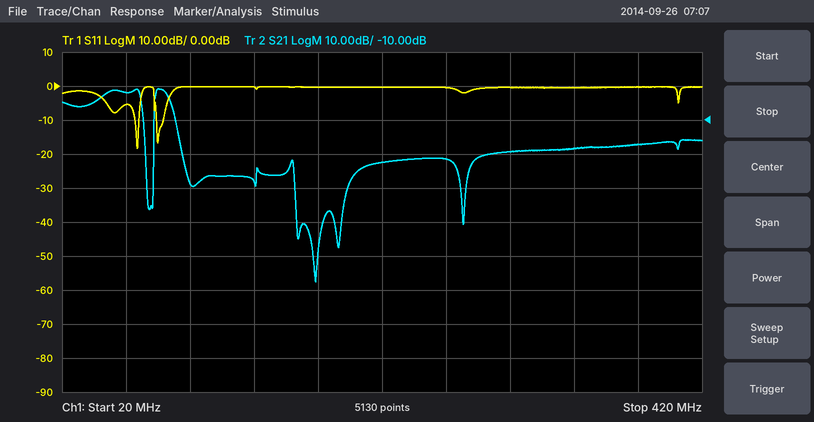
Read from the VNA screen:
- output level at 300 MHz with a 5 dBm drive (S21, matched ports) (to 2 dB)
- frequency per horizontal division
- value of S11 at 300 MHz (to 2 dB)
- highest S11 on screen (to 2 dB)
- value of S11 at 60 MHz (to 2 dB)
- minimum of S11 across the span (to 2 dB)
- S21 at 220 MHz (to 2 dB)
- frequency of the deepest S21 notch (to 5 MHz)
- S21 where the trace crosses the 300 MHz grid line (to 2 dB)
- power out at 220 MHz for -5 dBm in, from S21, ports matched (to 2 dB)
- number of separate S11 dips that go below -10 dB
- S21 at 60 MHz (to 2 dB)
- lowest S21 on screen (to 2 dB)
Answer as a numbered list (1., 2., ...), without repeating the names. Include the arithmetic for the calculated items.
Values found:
1. 5 dBm + (-20 dB) = -14 dBm
2. 40 MHz
3. 0 dB
4. 0 dB
5. -6 dB
6. -18 dB
7. -22 dB
8. 180 MHz
9. -20 dB
10. -5 dBm + (-22 dB) = -28 dBm
11. 2
12. -2 dB
13. -58 dB
